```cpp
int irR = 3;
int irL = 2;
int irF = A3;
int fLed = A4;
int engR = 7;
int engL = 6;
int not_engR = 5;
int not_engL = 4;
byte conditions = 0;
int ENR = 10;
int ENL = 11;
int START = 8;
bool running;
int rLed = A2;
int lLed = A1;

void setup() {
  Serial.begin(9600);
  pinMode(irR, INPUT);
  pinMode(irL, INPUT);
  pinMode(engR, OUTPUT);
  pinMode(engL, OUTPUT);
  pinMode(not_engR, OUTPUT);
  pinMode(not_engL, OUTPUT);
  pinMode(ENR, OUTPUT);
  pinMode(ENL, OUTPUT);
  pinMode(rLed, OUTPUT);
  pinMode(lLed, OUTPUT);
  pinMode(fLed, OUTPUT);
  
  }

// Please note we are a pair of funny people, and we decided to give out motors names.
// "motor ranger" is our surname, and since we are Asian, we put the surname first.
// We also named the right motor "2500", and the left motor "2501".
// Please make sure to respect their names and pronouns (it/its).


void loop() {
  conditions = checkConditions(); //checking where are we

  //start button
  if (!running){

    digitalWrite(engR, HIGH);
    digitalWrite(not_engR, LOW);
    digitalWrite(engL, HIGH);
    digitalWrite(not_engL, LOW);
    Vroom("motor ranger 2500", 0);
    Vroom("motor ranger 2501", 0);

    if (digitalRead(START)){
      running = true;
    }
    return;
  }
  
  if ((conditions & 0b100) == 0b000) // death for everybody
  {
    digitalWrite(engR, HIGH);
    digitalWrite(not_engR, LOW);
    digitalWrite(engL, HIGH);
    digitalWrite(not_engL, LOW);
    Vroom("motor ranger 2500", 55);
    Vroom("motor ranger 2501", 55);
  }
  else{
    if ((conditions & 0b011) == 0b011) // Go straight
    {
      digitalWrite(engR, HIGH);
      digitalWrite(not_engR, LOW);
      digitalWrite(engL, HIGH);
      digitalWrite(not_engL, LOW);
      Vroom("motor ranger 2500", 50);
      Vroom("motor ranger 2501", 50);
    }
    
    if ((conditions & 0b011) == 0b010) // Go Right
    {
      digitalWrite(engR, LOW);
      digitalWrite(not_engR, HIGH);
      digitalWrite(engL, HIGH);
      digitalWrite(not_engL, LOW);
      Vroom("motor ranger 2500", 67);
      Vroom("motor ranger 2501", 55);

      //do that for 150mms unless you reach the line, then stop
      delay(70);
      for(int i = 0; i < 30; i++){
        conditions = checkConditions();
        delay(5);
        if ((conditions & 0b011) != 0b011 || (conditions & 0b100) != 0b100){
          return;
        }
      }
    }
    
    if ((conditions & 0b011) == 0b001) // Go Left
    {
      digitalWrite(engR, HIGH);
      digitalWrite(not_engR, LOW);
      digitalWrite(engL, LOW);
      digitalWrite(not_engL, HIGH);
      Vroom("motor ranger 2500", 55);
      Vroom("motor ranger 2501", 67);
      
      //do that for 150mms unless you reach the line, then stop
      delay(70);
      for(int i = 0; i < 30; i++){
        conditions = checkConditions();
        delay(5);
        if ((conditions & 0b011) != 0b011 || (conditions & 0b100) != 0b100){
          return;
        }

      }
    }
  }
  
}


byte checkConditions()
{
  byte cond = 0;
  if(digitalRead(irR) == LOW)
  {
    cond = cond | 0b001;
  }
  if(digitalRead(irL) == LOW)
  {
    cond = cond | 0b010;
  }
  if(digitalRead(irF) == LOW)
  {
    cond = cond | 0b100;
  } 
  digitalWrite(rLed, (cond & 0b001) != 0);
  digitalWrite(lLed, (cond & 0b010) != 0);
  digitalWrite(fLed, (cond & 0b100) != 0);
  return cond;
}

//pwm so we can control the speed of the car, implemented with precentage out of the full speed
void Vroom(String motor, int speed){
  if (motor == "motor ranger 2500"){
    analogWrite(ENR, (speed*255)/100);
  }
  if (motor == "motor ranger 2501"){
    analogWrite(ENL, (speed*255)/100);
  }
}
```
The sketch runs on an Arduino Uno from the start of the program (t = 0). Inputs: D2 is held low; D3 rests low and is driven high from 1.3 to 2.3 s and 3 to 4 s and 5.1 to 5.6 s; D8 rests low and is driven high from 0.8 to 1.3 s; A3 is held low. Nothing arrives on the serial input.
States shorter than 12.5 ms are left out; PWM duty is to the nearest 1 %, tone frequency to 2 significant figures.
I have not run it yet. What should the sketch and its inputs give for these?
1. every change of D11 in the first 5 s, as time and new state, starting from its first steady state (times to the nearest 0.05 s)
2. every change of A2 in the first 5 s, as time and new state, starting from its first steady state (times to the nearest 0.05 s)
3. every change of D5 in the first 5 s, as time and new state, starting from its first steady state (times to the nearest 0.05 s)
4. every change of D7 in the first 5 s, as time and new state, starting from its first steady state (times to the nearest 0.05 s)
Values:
0 s low; 0.8 s PWM 50 %; 1.3 s PWM 55 %; 2.5 s PWM 50 %; 3 s PWM 55 %; 4.2 s PWM 50 %
0 s high; 1.3 s low; 2.35 s high; 3 s low; 4.05 s high
0 s low; 1.3 s high; 2.5 s low; 3 s high; 4.2 s low
0 s high; 1.3 s low; 2.5 s high; 3 s low; 4.2 s high
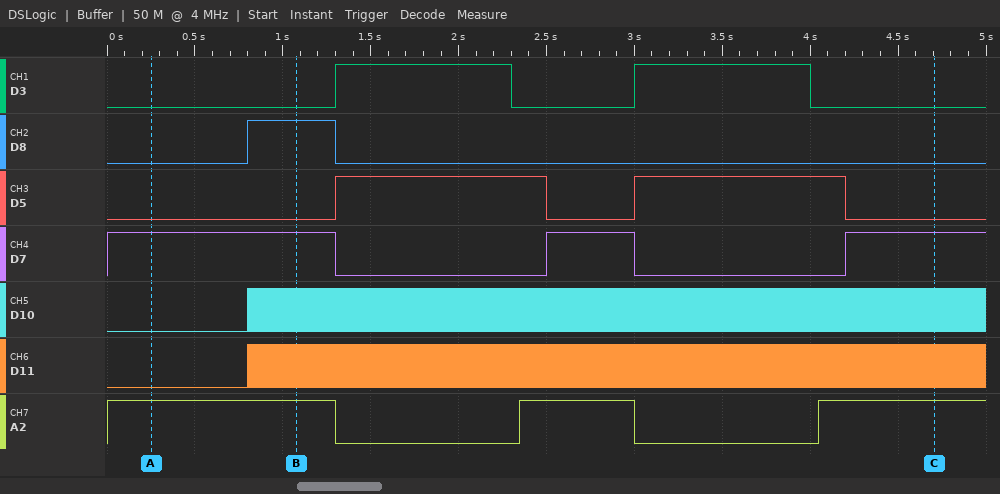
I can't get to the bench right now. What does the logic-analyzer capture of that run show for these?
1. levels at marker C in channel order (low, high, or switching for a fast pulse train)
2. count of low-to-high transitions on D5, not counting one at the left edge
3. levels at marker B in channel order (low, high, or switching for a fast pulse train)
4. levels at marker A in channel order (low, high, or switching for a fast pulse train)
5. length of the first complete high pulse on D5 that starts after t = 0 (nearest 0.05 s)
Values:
D3 low, D8 low, D5 low, D7 high, D10 switching, D11 switching, A2 high
2
D3 low, D8 high, D5 low, D7 high, D10 switching, D11 switching, A2 high
D3 low, D8 low, D5 low, D7 high, D10 low, D11 low, A2 high
1.20 s
